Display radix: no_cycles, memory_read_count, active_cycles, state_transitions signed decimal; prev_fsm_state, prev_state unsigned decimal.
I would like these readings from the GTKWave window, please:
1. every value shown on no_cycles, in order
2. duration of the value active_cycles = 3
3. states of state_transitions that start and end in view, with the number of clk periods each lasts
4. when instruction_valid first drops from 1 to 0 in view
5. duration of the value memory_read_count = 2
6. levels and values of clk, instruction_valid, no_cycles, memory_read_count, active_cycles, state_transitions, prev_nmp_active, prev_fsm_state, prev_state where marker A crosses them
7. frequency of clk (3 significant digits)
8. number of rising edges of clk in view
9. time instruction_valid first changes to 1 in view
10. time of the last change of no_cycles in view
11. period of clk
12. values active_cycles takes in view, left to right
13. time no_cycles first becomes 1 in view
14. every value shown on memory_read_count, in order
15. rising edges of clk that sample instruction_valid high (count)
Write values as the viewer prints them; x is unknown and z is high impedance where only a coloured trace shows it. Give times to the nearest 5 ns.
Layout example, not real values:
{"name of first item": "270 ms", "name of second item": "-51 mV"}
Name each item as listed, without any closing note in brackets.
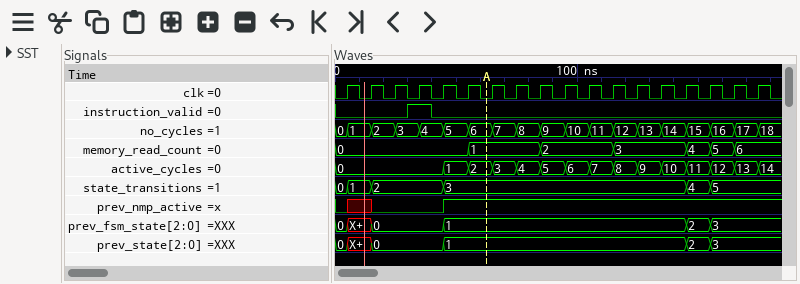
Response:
{"every value shown on no_cycles, in order": "0, 1, 2, 3, 4, 5, 6, 7, 8, 9, 10, 11, 12, 13, 14, 15, 16, 17, 18", "duration of the value active_cycles = 3": "10 ns", "states of state_transitions that start and end in view, with the number of clk periods each lasts": "1: 1, 2: 3, 3: 10, 4: 1", "when instruction_valid first drops from 1 to 0 in view": "40 ns", "duration of the value memory_read_count = 2": "30 ns", "levels and values of clk, instruction_valid, no_cycles, memory_read_count, active_cycles, state_transitions, prev_nmp_active, prev_fsm_state, prev_state where marker A crosses them": "clk=0, instruction_valid=0, no_cycles=6, memory_read_count=1, active_cycles=2, state_transitions=3, prev_nmp_active=1, prev_fsm_state=1, prev_state=1", "frequency of clk": "100 MHz", "number of rising edges of clk in view": "18", "time instruction_valid first changes to 1 in view": "30 ns", "time of the last change of no_cycles in view": "175 ns", "period of clk": "10 ns", "values active_cycles takes in view, left to right": "0, 1, 2, 3, 4, 5, 6, 7, 8, 9, 10, 11, 12, 13, 14", "time no_cycles first becomes 1 in view": "5 ns", "every value shown on memory_read_count, in order": "0, 1, 2, 3, 4, 5, 6", "rising edges of clk that sample instruction_valid high": "1"}
